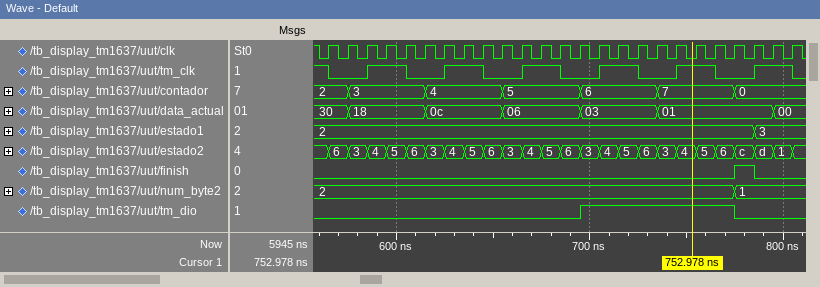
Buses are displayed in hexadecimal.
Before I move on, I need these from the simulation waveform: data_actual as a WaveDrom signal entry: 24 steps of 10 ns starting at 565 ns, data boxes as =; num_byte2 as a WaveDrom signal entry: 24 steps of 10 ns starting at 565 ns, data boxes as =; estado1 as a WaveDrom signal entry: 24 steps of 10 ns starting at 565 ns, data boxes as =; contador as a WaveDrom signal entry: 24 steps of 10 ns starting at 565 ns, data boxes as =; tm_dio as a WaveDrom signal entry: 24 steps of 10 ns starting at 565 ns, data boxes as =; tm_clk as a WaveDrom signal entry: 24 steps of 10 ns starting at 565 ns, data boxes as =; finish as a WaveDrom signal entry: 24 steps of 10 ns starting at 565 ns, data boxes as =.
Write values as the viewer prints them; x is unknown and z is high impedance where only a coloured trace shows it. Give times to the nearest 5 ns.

{name: 'data_actual', wave: '==...=...=...=...=.....=', data: '30 18 0c 06 03 01 00'}
{name: 'num_byte2', wave: '=....................=..', data: '2 1'}
{name: 'estado1', wave: '=.....................=.', data: '2 3'}
{name: 'contador', wave: '==...=...=...=...=...=..', data: '2 3 4 5 6 7 0'}
{name: 'tm_dio', wave: '0............1.......0..'}
{name: 'tm_clk', wave: '0.1.0.1.0.1.0.1.0.1.0.1.'}
{name: 'finish', wave: '0....................10.'}
